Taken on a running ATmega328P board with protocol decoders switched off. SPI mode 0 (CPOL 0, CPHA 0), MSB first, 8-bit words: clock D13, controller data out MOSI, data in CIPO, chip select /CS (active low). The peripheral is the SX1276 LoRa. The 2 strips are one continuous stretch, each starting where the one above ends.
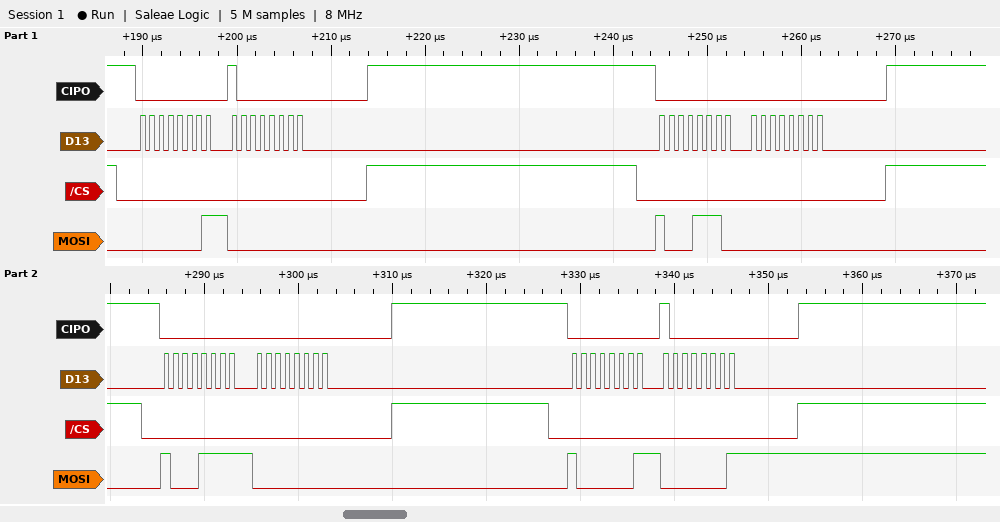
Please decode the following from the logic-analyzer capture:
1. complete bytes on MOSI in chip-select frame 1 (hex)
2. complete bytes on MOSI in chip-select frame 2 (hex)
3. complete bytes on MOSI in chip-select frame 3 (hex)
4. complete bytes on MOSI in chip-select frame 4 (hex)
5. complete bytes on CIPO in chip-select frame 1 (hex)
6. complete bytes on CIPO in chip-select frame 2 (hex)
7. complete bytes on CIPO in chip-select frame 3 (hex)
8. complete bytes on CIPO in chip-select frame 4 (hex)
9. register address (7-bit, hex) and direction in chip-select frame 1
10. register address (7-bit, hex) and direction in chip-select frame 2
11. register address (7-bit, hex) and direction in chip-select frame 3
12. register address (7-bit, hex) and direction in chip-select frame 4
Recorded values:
01 00
8E 00
8F 00
81 01
00 80
00 00
00 00
00 80
0x01 read
0x0E write
0x0F write
0x01 write
